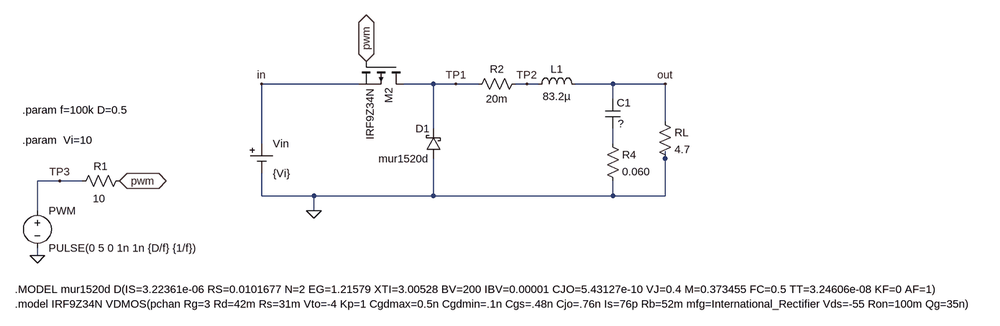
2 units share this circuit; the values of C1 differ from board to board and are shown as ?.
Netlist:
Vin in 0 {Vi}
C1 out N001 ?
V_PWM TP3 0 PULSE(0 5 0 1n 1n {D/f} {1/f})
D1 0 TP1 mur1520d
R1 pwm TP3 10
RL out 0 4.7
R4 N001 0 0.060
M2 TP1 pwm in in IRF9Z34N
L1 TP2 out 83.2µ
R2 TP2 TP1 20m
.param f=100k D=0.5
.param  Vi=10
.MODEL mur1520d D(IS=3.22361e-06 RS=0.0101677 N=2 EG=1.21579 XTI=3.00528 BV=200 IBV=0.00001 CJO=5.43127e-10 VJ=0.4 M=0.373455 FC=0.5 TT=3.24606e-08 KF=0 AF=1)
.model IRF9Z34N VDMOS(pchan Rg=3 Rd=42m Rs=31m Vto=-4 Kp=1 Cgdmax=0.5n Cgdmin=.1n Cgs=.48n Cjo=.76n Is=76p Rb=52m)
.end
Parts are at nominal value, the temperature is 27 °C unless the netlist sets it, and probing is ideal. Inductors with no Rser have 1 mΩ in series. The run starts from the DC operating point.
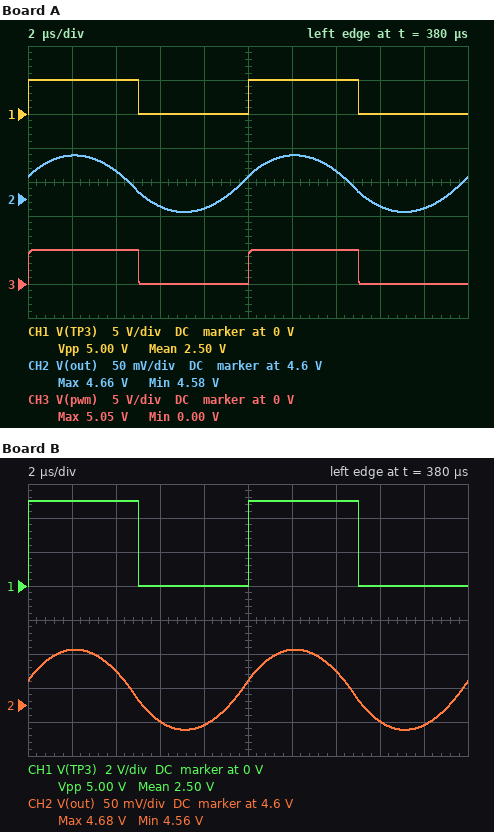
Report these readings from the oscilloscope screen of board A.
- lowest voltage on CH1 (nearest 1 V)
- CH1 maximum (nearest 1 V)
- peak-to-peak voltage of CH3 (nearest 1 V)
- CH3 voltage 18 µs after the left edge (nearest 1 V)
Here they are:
0 V
5 V
5 V
0 V
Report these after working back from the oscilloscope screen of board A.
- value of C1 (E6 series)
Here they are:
4.7 µF
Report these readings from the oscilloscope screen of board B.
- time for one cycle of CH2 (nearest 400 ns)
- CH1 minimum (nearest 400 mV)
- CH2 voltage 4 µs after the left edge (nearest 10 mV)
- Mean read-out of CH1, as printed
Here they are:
10.0 µs
0 V
4.65 V
2.50 V
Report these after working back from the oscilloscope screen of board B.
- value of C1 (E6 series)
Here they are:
3.3 µF
